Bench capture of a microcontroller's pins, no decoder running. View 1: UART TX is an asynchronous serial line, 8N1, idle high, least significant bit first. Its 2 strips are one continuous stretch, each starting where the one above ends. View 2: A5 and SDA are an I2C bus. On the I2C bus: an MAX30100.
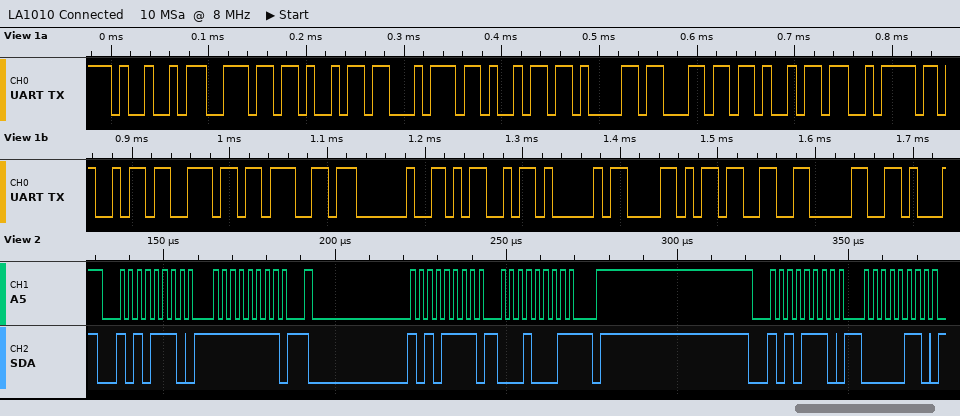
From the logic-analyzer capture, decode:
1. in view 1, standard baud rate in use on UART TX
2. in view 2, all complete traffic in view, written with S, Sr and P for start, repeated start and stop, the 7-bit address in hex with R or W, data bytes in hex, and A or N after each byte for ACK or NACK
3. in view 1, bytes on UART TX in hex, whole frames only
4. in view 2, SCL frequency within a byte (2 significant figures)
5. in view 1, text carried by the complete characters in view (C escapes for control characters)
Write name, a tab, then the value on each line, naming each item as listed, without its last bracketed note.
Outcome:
in view 1, standard baud rate in use on UART TX	115200 baud
in view 2, all complete traffic in view, written with S, Sr and P for start, repeated start and stop, the 7-bit address in hex with R or W, data bytes in hex, and A or N after each byte for ACK or NACK	S 57W A FF A Sr 57R A 11 N P S 57W A 06 A
in view 1, bytes on UART TX in hex, whole frames only	49 6E 69 74 69 61 6C 69 7A 69 6E 67 20 4D 41 58 33 30
in view 2, SCL frequency within a byte	400 kHz
in view 1, text carried by the complete characters in view	"Initializing MAX30"
